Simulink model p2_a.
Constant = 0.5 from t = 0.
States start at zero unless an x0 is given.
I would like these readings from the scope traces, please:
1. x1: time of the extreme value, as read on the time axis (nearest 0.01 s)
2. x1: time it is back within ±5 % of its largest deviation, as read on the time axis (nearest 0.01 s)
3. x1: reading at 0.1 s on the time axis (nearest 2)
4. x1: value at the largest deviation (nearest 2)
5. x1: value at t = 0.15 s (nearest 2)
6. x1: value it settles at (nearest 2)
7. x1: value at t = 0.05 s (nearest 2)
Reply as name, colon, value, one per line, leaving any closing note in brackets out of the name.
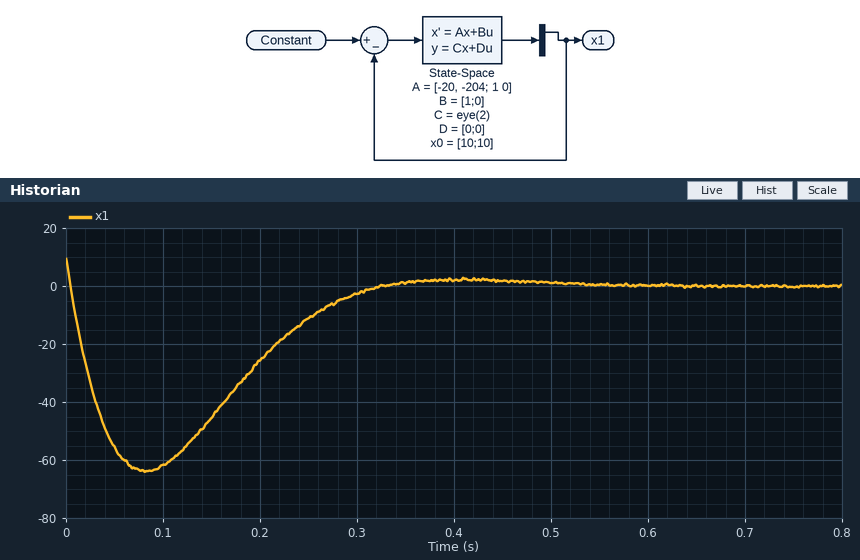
x1: time of the extreme value, as read on the time axis: 0.08 s
x1: time it is back within ±5 % of its largest deviation, as read on the time axis: 0.29 s
x1: reading at 0.1 s on the time axis: -62
x1: value at the largest deviation: -64
x1: value at t = 0.15 s: -46
x1: value it settles at: 0
x1: value at t = 0.05 s: -56
